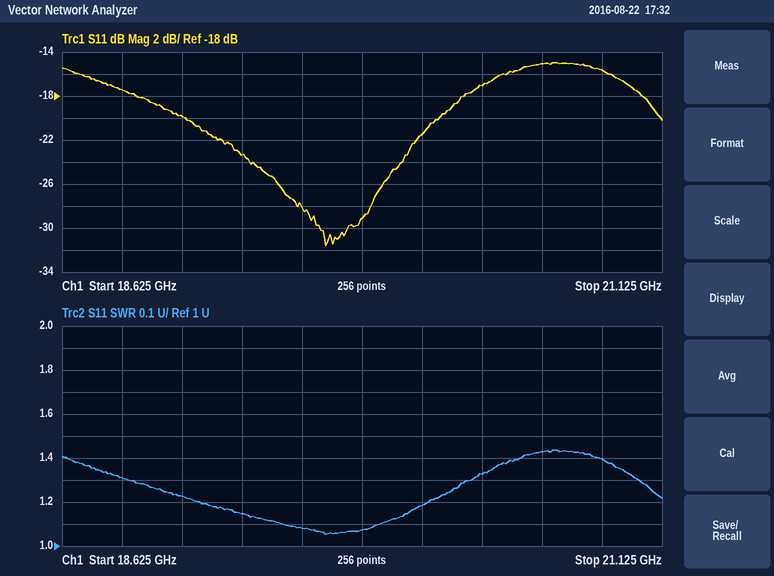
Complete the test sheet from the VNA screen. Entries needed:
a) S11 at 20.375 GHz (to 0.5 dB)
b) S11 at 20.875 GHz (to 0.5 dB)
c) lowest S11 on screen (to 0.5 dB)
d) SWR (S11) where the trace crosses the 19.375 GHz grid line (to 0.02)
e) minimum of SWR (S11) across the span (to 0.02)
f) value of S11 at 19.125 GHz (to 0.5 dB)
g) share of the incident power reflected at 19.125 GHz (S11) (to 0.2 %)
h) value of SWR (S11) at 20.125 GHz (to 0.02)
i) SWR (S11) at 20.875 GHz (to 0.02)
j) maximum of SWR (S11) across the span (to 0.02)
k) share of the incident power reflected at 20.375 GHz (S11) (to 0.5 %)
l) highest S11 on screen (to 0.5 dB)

-17.0 dB
-15.5 dB
-31.5 dB
1.14
1.06
-20.0 dB
1.0 %
1.18
1.40
1.44
2.0 %
-15.0 dB
